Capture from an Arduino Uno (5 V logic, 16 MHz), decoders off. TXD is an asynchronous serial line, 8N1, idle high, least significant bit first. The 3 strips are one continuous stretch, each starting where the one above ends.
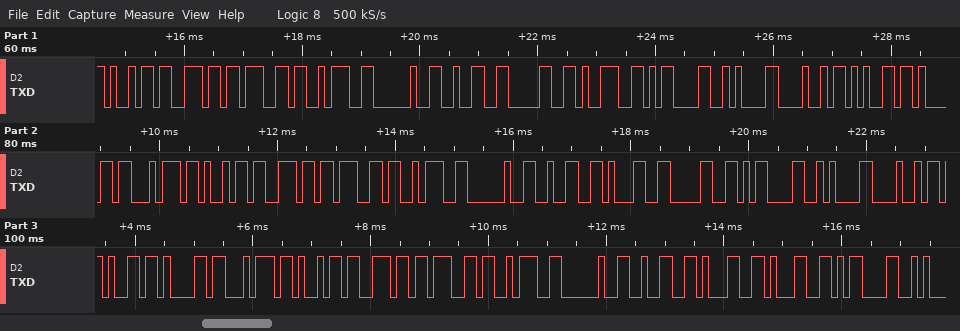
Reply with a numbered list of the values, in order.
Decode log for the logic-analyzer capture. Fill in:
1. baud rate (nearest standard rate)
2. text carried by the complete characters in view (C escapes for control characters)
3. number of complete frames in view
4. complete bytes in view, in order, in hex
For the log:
1. 9600 baud
2. "ing: 209\r\nHeating: 210\r\nHeating: 211\r"
3. 37
4. 0x69 0x6E 0x67 0x3A 0x20 0x32 0x30 0x39 0x0D 0x0A 0x48 0x65 0x61 0x74 0x69 0x6E 0x67 0x3A 0x20 0x32 0x31 0x30 0x0D 0x0A 0x48 0x65 0x61 0x74 0x69 0x6E 0x67 0x3A 0x20 0x32 0x31 0x31 0x0D
